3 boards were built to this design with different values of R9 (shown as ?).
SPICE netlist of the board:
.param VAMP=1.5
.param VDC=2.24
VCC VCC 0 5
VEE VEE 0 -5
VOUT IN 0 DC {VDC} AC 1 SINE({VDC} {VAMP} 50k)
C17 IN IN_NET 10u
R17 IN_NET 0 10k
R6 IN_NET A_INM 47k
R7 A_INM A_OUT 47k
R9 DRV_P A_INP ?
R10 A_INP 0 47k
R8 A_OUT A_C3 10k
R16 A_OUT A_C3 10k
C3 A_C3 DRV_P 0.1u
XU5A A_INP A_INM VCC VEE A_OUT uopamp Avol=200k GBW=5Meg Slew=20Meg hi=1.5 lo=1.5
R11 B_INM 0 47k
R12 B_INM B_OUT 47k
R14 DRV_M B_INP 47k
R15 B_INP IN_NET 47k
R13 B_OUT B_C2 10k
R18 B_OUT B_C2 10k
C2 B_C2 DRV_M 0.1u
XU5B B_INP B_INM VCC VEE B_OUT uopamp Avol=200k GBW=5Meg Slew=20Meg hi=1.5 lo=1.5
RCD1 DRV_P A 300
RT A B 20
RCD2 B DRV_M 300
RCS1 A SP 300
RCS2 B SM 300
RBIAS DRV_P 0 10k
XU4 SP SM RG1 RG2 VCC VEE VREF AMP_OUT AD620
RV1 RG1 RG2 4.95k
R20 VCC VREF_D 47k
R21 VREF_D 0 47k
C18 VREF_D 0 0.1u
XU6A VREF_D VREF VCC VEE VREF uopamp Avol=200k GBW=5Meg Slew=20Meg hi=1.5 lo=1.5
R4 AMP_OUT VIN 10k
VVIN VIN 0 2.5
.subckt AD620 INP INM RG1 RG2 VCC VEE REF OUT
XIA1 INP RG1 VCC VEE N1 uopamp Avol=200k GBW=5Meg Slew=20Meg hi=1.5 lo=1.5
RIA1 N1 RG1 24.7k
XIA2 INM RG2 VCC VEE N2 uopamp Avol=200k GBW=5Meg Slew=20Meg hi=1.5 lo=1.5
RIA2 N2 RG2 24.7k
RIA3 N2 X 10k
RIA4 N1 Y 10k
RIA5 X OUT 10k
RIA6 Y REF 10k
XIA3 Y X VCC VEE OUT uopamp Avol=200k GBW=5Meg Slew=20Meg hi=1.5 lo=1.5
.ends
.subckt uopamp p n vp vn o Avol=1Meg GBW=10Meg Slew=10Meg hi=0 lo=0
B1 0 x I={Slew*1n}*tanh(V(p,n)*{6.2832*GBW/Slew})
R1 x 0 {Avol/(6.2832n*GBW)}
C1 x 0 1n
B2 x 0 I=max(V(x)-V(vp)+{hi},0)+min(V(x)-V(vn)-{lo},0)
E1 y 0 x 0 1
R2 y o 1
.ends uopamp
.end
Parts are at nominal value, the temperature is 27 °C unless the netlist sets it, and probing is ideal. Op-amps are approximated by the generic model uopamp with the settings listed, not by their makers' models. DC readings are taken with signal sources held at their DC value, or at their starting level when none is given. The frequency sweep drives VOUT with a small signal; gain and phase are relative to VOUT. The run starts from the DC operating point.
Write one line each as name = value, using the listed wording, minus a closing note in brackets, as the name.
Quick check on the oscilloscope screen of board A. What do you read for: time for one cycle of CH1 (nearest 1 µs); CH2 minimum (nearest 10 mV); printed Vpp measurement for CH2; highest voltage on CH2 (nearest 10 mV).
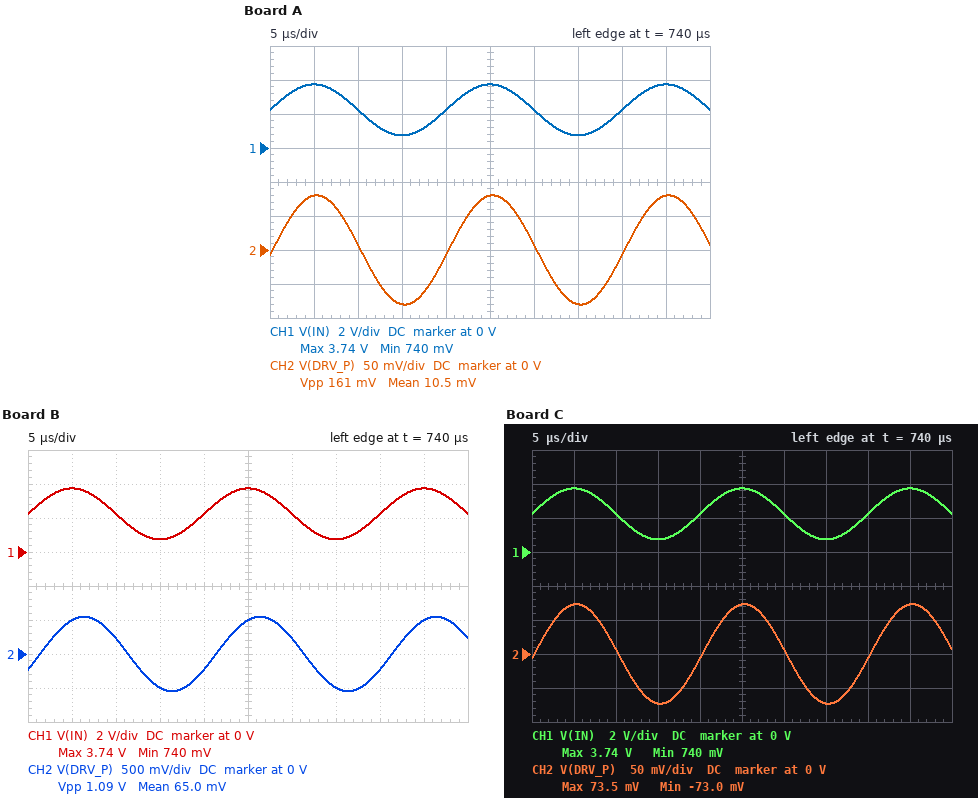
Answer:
time for one cycle of CH1 = 20 µs
CH2 minimum = -80 mV
printed Vpp measurement for CH2 = 161 mV
highest voltage on CH2 = 80 mV
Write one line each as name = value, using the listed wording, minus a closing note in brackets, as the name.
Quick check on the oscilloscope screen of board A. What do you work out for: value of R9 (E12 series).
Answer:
value of R9 = 82 kΩ
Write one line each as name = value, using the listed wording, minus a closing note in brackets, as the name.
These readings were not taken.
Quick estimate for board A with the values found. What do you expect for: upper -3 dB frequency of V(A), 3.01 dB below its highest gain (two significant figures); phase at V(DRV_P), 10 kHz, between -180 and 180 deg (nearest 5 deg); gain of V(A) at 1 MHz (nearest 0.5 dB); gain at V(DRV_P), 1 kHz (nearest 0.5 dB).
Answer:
upper -3 dB frequency of V(A), 3.01 dB below its highest gain = 790 kHz
phase at V(DRV_P), 10 kHz, between -180 and 180 deg = 0 deg
gain of V(A) at 1 MHz = -23.0 dB
gain at V(DRV_P), 1 kHz = -25.0 dB
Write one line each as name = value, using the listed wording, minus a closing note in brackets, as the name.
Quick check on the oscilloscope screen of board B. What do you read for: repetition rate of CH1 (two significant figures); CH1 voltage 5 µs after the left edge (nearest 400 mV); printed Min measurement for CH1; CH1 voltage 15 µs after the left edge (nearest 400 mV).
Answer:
repetition rate of CH1 = 50 kHz
CH1 voltage 5 µs after the left edge = 3.6 V
printed Min measurement for CH1 = 740 mV
CH1 voltage 15 µs after the left edge = 800 mV
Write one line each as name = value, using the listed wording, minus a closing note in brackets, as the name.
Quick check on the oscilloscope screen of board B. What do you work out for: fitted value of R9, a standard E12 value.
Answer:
fitted value of R9, a standard E12 value = 15 kΩ
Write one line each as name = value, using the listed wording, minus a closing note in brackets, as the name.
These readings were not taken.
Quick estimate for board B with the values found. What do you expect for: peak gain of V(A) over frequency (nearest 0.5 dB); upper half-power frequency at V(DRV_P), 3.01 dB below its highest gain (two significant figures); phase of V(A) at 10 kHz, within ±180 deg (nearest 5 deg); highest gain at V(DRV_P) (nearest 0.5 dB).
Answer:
peak gain of V(A) over frequency = -7.0 dB
upper half-power frequency at V(DRV_P), 3.01 dB below its highest gain = 110 kHz
phase of V(A) at 10 kHz, within ±180 deg = 0 deg
highest gain at V(DRV_P) = -8.0 dB
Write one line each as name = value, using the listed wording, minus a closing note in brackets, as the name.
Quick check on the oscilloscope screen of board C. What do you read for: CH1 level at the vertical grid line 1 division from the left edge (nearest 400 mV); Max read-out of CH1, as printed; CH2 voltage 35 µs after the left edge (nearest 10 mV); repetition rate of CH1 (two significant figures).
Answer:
CH1 level at the vertical grid line 1 division from the left edge = 3.6 V
Max read-out of CH1, as printed = 3.74 V
CH2 voltage 35 µs after the left edge = -70 mV
repetition rate of CH1 = 50 kHz
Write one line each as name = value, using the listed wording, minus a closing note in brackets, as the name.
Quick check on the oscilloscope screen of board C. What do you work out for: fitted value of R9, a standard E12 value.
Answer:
fitted value of R9, a standard E12 value = 100 kΩ
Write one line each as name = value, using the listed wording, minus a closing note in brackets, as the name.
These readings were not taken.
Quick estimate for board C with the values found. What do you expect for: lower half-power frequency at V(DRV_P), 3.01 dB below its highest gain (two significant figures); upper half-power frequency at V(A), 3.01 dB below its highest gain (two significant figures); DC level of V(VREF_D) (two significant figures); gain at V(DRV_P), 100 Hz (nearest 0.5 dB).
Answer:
lower half-power frequency at V(DRV_P), 3.01 dB below its highest gain = 2.0 Hz
upper half-power frequency at V(A), 3.01 dB below its highest gain = 850 kHz
DC level of V(VREF_D) = 2.5 V
gain at V(DRV_P), 100 Hz = -21.5 dB
